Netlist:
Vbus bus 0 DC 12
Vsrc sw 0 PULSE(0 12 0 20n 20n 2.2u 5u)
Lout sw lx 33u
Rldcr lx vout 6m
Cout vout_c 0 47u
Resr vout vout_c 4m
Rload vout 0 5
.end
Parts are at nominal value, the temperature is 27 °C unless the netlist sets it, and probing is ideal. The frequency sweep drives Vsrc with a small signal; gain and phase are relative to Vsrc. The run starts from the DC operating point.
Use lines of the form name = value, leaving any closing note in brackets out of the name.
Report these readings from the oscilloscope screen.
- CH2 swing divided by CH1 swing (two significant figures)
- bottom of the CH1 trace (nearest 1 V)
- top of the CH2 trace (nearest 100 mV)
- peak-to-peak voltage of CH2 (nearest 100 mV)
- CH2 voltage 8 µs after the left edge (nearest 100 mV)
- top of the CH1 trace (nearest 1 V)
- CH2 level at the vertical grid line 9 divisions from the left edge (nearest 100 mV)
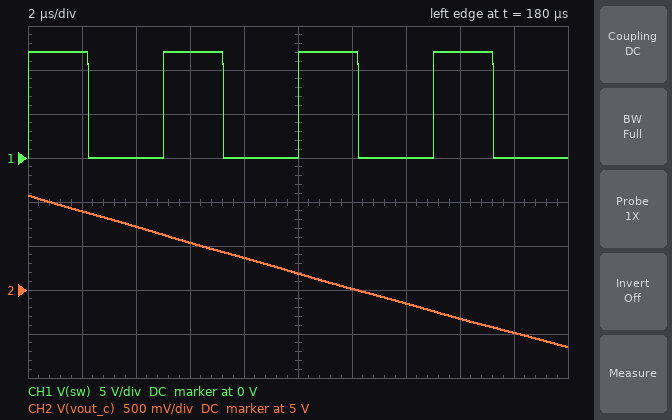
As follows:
CH2 swing divided by CH1 swing = 0.14
bottom of the CH1 trace = 0 V
top of the CH2 trace = 6.1 V
peak-to-peak voltage of CH2 = 1.7 V
CH2 voltage 8 µs after the left edge = 5.4 V
top of the CH1 trace = 12 V
CH2 level at the vertical grid line 9 divisions from the left edge = 4.5 V
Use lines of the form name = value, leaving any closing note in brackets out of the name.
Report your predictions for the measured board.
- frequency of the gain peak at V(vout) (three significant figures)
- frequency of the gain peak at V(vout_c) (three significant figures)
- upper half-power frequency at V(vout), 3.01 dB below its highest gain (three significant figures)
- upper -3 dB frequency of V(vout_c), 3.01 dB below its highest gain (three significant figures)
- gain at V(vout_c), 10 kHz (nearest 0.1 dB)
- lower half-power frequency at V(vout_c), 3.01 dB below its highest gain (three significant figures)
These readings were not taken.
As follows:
frequency of the gain peak at V(vout) = 4.01 kHz
frequency of the gain peak at V(vout_c) = 4.01 kHz
upper half-power frequency at V(vout), 3.01 dB below its highest gain = 4.36 kHz
upper -3 dB frequency of V(vout_c), 3.01 dB below its highest gain = 4.36 kHz
gain at V(vout_c), 10 kHz = -14.2 dB
lower half-power frequency at V(vout_c), 3.01 dB below its highest gain = 3.63 kHz
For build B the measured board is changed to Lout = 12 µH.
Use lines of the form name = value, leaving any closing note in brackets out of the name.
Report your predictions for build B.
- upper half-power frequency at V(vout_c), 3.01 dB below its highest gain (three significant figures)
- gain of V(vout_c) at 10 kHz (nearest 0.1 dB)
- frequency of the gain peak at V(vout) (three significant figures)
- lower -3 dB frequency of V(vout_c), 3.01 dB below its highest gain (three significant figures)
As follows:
upper half-power frequency at V(vout_c), 3.01 dB below its highest gain = 7.07 kHz
gain of V(vout_c) at 10 kHz = -1.9 dB
frequency of the gain peak at V(vout) = 6.68 kHz
lower -3 dB frequency of V(vout_c), 3.01 dB below its highest gain = 6.26 kHz
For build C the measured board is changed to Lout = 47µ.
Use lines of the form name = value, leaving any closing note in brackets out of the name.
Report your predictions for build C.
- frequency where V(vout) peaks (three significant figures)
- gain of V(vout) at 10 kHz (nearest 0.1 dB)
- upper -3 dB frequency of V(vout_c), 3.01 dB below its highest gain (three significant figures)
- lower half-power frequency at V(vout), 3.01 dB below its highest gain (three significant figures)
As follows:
frequency where V(vout) peaks = 3.35 kHz
gain of V(vout) at 10 kHz = -17.8 dB
upper -3 dB frequency of V(vout_c), 3.01 dB below its highest gain = 3.69 kHz
lower half-power frequency at V(vout), 3.01 dB below its highest gain = 2.97 kHz
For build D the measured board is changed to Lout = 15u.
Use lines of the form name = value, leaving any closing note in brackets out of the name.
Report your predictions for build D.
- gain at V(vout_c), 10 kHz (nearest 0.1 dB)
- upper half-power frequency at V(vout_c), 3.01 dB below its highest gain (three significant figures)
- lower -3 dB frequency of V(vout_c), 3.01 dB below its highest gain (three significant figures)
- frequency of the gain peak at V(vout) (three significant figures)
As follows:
gain at V(vout_c), 10 kHz = -5.1 dB
upper half-power frequency at V(vout_c), 3.01 dB below its highest gain = 6.35 kHz
lower -3 dB frequency of V(vout_c), 3.01 dB below its highest gain = 5.56 kHz
frequency of the gain peak at V(vout) = 5.97 kHz
